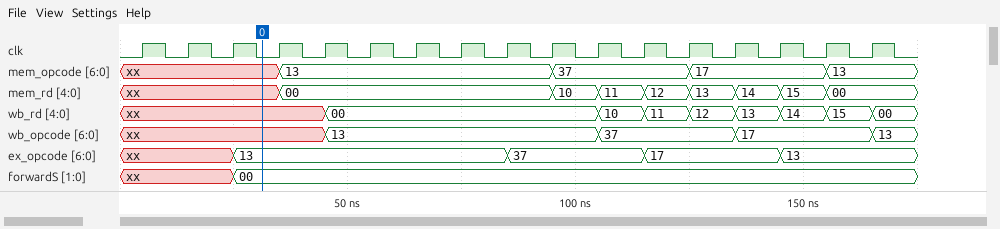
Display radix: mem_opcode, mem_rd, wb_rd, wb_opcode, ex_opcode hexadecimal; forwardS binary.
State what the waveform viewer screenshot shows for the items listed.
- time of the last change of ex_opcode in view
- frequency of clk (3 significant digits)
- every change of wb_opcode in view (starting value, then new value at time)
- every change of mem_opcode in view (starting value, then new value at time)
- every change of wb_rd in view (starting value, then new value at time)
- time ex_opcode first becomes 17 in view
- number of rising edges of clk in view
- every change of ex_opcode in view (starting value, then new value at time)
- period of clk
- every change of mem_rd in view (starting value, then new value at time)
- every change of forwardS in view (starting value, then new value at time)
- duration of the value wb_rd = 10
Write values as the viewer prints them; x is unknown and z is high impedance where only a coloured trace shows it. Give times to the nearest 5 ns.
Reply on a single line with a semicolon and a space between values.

145 ns; 100 MHz; xx, 13 at 45 ns, 37 at 105 ns, 17 at 135 ns, 13 at 165 ns; xx, 13 at 35 ns, 37 at 95 ns, 17 at 125 ns, 13 at 155 ns; xx, 00 at 45 ns, 10 at 105 ns, 11 at 115 ns, 12 at 125 ns, 13 at 135 ns, 14 at 145 ns, 15 at 155 ns, 00 at 165 ns; 115 ns; 17; xx, 13 at 25 ns, 37 at 85 ns, 17 at 115 ns, 13 at 145 ns; 10 ns; xx, 00 at 35 ns, 10 at 95 ns, 11 at 105 ns, 12 at 115 ns, 13 at 125 ns, 14 at 135 ns, 15 at 145 ns, 00 at 155 ns; xx, 00 at 25 ns; 10 ns
